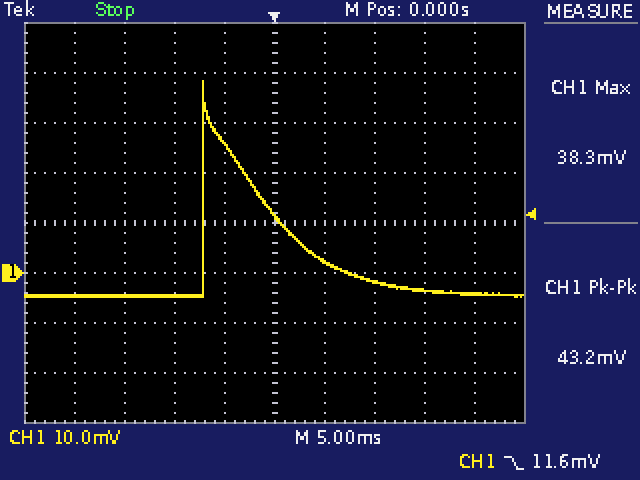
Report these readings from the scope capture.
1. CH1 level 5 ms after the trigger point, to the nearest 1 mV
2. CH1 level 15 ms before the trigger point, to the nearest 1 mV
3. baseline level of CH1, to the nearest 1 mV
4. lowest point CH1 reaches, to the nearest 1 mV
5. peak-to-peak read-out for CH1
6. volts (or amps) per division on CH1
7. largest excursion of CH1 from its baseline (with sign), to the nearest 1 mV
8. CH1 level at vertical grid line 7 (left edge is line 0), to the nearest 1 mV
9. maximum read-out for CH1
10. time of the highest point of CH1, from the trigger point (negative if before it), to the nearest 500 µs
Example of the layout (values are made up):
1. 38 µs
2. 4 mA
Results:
1. 2 mV
2. -5 mV
3. -5 mV
4. -5 mV
5. 43.2 mV
6. 10 mV
7. +43 mV
8. -2 mV
9. 38.3 mV
10. -7.0 ms
